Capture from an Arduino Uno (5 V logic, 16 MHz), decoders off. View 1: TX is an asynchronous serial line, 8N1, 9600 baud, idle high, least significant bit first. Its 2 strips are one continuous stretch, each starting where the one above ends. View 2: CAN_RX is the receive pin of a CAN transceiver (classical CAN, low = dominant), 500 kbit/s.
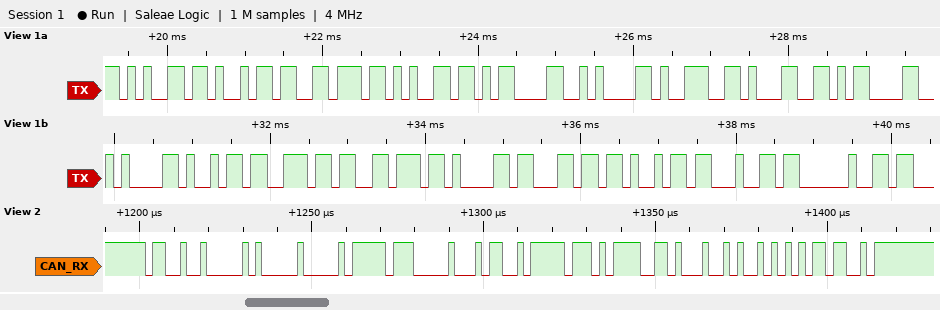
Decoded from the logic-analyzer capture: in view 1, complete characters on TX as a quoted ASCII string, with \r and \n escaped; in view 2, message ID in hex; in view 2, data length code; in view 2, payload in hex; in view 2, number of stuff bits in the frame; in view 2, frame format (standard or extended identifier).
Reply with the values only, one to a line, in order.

"eive\r\n91\r\ninvalid "
0x648
8
00 FF 00 B2 FF 5E 68 94
6
standard
